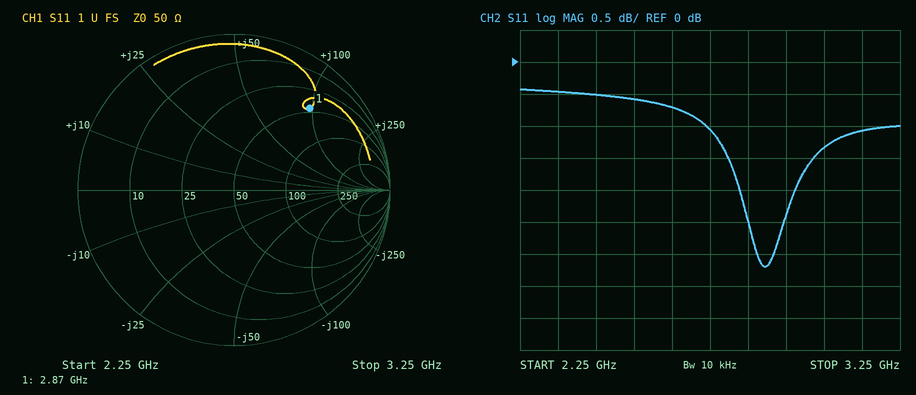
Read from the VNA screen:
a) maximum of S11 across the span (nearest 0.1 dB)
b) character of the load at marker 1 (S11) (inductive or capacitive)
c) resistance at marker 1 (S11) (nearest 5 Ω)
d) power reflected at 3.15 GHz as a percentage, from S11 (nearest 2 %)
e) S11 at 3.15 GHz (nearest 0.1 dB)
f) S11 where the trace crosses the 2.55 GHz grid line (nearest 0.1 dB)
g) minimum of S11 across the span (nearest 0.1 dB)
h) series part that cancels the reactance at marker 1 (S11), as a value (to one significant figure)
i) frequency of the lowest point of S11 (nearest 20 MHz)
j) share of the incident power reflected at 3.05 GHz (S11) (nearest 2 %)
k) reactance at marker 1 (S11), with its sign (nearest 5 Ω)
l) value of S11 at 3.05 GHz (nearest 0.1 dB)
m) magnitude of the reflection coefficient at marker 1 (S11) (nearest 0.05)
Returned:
-0.4 dB
inductive
45 Ω
78 %
-1.1 dB
-0.6 dB
-3.2 dB
600 fF
2.90 GHz
74 %
+95 Ω
-1.3 dB
0.70
